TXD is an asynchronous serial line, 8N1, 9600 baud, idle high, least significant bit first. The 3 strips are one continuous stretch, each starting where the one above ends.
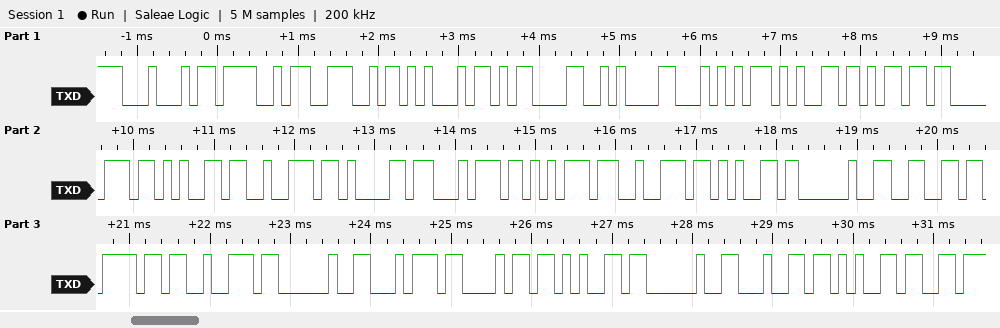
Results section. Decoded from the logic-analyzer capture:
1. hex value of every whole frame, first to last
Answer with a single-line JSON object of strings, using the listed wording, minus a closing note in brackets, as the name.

{"hex value of every whole frame, first to last": "44 4F 4E 45 0D 0A 54 65 6D 70 65 72 61 74 75 72 65 20 66 6F 72 20 74 68 65 20 64 65"}
